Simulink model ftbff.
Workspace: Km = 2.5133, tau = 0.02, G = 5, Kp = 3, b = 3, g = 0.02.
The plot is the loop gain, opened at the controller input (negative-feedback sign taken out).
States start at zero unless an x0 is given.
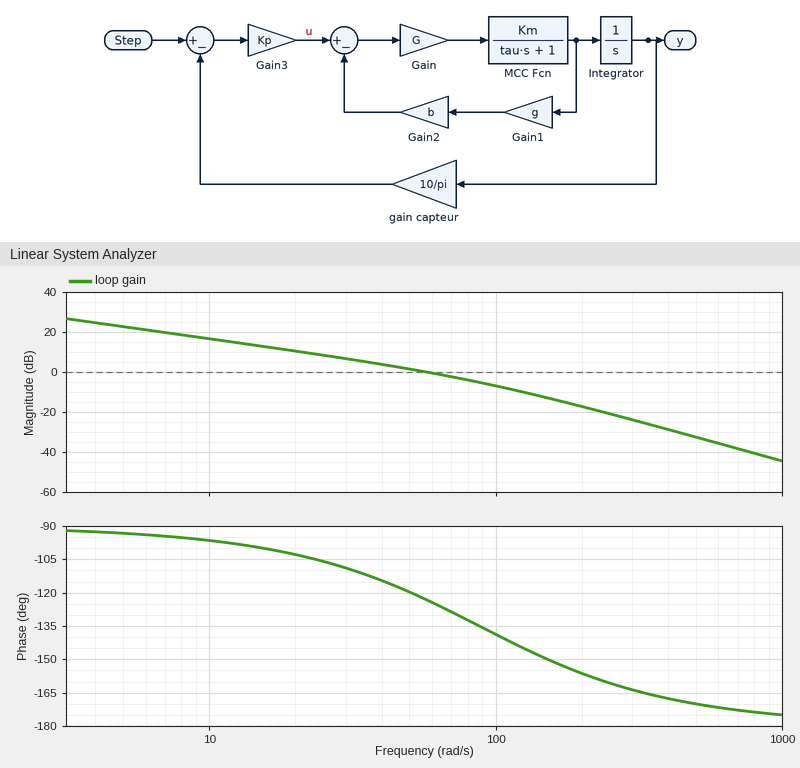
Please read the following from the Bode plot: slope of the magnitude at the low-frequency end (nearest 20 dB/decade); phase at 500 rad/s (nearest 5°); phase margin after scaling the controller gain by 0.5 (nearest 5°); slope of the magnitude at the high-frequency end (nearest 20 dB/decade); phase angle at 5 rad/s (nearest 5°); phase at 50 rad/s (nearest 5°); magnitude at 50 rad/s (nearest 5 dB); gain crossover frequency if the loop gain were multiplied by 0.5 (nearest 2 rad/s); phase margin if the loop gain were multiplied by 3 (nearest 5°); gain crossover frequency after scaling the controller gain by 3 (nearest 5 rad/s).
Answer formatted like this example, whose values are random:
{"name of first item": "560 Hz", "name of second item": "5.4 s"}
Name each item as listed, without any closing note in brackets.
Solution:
{"slope of the magnitude at the low-frequency end": "-20 dB/decade", "phase at 500 rad/s": "-170°", "phase margin after scaling the controller gain by 0.5": "70°", "slope of the magnitude at the high-frequency end": "-40 dB/decade", "phase angle at 5 rad/s": "-95°", "phase at 50 rad/s": "-120°", "magnitude at 50 rad/s": "0 dB", "gain crossover frequency if the loop gain were multiplied by 0.5": "32 rad/s", "phase margin if the loop gain were multiplied by 3": "35°", "gain crossover frequency after scaling the controller gain by 3": "120 rad/s"}
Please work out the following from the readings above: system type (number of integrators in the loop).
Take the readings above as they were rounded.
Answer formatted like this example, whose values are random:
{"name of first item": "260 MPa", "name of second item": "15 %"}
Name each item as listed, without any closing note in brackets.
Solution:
{"system type": "1"}
